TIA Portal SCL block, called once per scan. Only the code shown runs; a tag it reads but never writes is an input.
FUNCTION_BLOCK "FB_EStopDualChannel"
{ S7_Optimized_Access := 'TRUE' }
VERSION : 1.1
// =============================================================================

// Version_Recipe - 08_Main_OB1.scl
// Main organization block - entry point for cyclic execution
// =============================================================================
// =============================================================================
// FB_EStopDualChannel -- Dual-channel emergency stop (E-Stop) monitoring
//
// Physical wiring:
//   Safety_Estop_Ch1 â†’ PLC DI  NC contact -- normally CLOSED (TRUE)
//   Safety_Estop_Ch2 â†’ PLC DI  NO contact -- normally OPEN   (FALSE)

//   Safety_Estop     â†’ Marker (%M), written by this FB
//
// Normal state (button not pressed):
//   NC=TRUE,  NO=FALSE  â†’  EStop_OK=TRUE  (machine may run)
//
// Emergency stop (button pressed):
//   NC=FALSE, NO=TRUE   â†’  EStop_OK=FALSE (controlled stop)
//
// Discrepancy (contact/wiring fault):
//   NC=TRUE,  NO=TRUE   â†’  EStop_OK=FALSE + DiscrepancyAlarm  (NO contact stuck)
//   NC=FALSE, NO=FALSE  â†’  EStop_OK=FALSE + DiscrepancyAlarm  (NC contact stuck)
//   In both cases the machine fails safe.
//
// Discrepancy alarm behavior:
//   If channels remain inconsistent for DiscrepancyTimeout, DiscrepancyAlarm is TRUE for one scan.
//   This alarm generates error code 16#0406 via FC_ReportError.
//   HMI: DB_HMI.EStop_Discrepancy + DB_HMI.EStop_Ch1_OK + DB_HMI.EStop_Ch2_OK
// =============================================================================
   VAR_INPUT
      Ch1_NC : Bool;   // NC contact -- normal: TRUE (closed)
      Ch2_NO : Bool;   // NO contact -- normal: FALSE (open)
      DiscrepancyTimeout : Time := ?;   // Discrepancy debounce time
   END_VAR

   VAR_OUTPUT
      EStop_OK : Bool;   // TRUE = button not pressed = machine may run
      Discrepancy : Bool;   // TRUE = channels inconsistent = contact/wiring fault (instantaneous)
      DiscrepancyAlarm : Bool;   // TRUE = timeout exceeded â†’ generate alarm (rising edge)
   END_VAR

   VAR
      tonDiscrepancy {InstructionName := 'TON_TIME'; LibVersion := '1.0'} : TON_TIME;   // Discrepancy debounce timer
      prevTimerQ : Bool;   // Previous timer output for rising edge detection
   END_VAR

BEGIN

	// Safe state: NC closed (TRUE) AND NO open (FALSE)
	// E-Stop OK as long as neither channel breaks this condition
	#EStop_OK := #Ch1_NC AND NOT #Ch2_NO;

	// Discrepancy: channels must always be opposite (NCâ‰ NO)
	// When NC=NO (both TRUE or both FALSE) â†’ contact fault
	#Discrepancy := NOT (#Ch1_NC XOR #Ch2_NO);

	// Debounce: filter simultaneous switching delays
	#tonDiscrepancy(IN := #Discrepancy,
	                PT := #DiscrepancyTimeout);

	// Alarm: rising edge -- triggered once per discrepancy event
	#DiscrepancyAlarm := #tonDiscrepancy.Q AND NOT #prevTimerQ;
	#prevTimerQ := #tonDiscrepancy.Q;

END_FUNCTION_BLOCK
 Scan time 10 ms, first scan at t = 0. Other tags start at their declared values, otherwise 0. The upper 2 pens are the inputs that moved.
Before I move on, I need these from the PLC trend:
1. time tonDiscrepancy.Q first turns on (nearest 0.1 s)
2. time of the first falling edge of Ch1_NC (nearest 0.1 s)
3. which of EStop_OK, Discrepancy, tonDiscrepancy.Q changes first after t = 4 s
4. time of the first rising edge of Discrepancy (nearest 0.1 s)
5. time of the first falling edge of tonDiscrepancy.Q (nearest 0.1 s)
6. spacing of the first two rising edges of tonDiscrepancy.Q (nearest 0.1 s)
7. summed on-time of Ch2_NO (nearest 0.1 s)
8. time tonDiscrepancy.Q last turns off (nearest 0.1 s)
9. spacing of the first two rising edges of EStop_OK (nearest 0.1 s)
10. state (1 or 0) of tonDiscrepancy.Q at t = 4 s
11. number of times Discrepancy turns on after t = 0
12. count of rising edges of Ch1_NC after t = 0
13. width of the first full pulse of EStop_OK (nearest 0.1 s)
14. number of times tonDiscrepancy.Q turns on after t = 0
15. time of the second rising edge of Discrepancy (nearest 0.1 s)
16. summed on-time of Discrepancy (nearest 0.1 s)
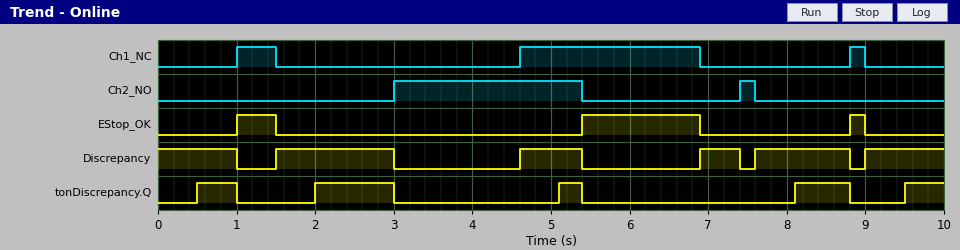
0.5 s
1.5 s
Discrepancy
1.5 s
1.0 s
1.5 s
2.6 s
8.8 s
4.4 s
0
5
3
0.5 s
5
4.6 s
6.0 s
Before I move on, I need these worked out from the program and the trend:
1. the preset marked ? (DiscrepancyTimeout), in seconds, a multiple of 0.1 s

0.5 s
